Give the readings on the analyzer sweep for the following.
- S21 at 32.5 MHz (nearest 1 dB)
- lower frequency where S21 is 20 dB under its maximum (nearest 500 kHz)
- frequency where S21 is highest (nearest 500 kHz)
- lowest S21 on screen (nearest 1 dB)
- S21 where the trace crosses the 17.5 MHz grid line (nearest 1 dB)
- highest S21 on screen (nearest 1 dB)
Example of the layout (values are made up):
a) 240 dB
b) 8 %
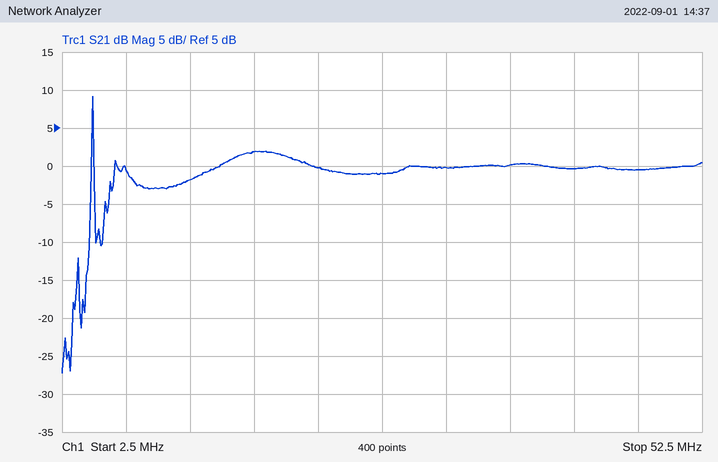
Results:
a) 0 dB
b) 4.5 MHz
c) 5.0 MHz
d) -27 dB
e) 2 dB
f) 9 dB
